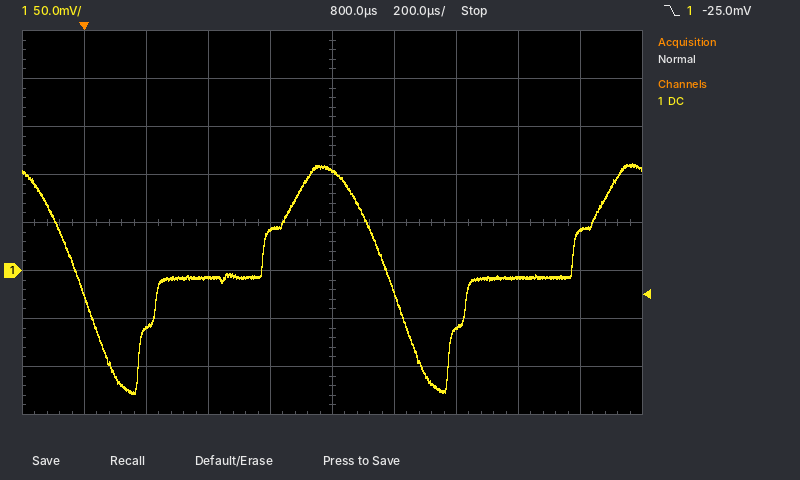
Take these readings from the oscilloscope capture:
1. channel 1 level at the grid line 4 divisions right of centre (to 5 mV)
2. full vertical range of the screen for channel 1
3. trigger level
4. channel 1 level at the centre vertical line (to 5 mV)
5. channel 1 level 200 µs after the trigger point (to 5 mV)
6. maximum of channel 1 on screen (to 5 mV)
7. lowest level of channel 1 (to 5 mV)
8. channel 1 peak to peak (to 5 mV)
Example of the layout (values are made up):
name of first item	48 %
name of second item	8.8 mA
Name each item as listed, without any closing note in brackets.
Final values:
channel 1 level at the grid line 4 divisions right of centre	40 mV
full vertical range of the screen for channel 1	400 mV
trigger level	-25.0 mV
channel 1 level at the centre vertical line	105 mV
channel 1 level 200 µs after the trigger point	-60 mV
maximum of channel 1 on screen	110 mV
lowest level of channel 1	-130 mV
channel 1 peak to peak	240 mV
